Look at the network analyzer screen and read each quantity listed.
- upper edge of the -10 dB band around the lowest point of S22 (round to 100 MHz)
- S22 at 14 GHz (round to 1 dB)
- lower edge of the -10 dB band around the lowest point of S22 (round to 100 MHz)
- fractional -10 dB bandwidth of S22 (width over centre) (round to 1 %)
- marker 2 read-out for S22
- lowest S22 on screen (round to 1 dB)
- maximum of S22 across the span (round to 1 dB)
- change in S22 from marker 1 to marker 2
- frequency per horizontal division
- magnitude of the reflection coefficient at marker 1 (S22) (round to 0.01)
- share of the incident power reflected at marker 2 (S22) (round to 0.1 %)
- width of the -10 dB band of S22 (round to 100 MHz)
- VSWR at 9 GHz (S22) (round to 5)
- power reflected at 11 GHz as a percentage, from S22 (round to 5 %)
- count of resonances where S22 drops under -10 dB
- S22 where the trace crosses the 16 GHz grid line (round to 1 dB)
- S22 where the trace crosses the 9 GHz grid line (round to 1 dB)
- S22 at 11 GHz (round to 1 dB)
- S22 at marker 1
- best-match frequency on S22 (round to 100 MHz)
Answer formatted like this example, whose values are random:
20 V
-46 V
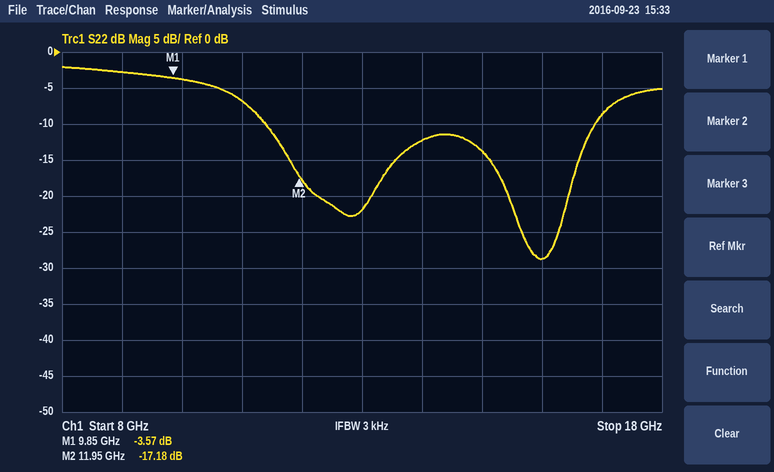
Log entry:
16.9 GHz
-12 dB
11.4 GHz
39 %
-17.18 dB
-29 dB
-2 dB
-13.61 dB
1 GHz
0.66
1.9 %
5.5 GHz
5
20 %
2
-29 dB
-3 dB
-7 dB
-3.57 dB
16.0 GHz
